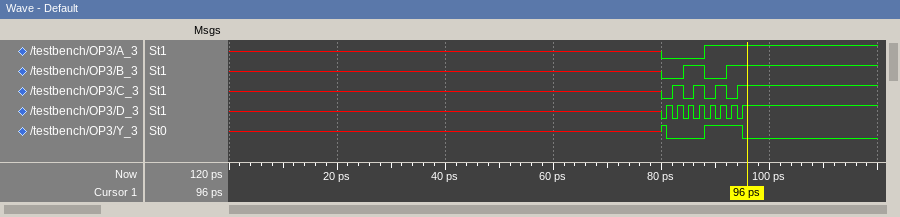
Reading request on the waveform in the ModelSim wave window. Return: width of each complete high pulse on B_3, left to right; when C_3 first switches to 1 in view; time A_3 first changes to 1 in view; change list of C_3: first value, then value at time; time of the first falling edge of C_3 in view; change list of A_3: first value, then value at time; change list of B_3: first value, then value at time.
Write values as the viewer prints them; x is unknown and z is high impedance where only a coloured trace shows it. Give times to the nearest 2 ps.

4 ps
82 ps
88 ps
x, 0 at 80 ps, 1 at 82 ps, 0 at 84 ps, 1 at 86 ps, 0 at 88 ps, 1 at 90 ps, 0 at 92 ps, 1 at 94 ps
84 ps
x, 0 at 80 ps, 1 at 88 ps
x, 0 at 80 ps, 1 at 84 ps, 0 at 88 ps, 1 at 92 ps
